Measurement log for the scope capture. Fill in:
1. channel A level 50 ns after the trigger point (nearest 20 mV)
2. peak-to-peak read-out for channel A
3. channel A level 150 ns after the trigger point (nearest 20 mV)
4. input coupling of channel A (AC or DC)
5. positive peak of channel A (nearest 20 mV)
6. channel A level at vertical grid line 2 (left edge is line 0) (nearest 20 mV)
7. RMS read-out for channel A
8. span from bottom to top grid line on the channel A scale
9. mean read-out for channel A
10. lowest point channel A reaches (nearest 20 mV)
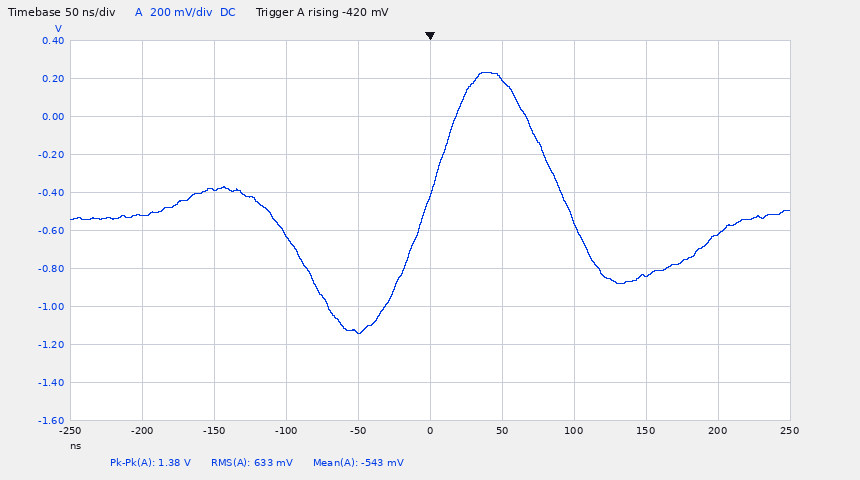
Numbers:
200 mV
1.38 V
-840 mV
DC
240 mV
-380 mV
633 mV
2 V
-543 mV
-1.14 V
